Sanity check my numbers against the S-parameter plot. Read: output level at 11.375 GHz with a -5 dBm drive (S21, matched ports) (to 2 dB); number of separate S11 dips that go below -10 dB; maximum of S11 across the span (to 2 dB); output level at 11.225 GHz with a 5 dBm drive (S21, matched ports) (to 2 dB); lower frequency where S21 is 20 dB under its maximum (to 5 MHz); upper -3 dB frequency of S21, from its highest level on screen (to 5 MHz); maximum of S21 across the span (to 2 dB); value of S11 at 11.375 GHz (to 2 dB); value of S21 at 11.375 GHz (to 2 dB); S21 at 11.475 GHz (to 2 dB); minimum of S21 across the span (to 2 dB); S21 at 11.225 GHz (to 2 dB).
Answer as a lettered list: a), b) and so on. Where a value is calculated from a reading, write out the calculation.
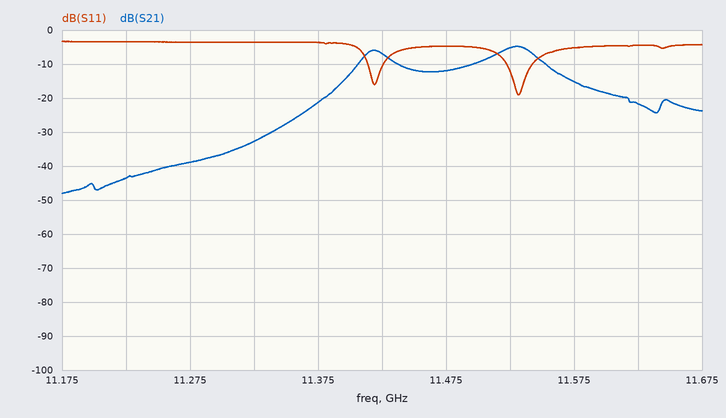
a) -5 dBm + (-22 dB) = -26 dBm
b) 2
c) -4 dB
d) 5 dBm + (-44 dB) = -38 dBm
e) 11.360 GHz
f) 11.545 GHz
g) -4 dB
h) -4 dB
i) -22 dB
j) -12 dB
k) -48 dB
l) -44 dB
